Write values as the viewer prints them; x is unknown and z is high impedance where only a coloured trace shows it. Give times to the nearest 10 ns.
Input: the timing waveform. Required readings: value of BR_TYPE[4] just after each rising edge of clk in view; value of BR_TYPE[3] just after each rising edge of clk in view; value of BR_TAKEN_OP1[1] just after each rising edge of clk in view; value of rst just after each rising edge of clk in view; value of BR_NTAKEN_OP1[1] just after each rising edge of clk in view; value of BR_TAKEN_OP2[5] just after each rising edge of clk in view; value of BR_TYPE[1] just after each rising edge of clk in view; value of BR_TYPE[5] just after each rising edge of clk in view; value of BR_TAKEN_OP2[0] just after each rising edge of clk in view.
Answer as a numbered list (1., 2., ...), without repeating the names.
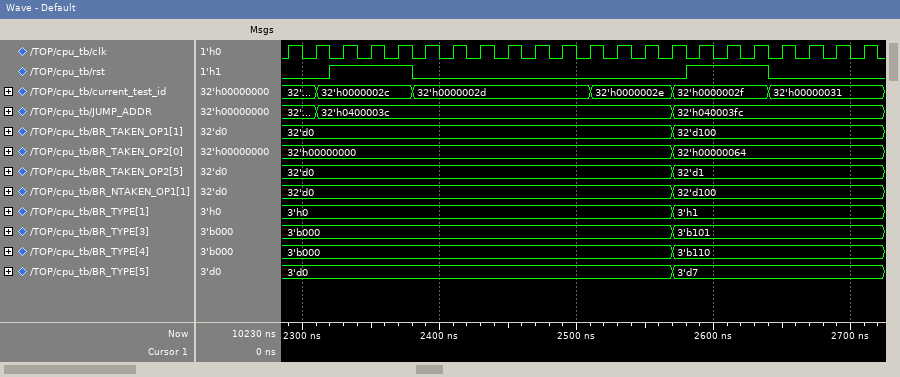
1. 3'b000, 3'b000, 3'b000, 3'b000, 3'b000, 3'b000, 3'b000, 3'b000, 3'b000, 3'b000, 3'b000, 3'b000, 3'b000, 3'b000, 3'b110, 3'b110, 3'b110, 3'b110, 3'b110, 3'b110, 3'b110, 3'b110
2. 3'b000, 3'b000, 3'b000, 3'b000, 3'b000, 3'b000, 3'b000, 3'b000, 3'b000, 3'b000, 3'b000, 3'b000, 3'b000, 3'b000, 3'b101, 3'b101, 3'b101, 3'b101, 3'b101, 3'b101, 3'b101, 3'b101
3. 32'd0, 32'd0, 32'd0, 32'd0, 32'd0, 32'd0, 32'd0, 32'd0, 32'd0, 32'd0, 32'd0, 32'd0, 32'd0, 32'd0, 32'd100, 32'd100, 32'd100, 32'd100, 32'd100, 32'd100, 32'd100, 32'd100
4. 0 0 1 1 1 0 0 0 0 0 0 0 0 0 0 1 1 1 0 0 0 0
5. 32'd0, 32'd0, 32'd0, 32'd0, 32'd0, 32'd0, 32'd0, 32'd0, 32'd0, 32'd0, 32'd0, 32'd0, 32'd0, 32'd0, 32'd100, 32'd100, 32'd100, 32'd100, 32'd100, 32'd100, 32'd100, 32'd100
6. 32'd0, 32'd0, 32'd0, 32'd0, 32'd0, 32'd0, 32'd0, 32'd0, 32'd0, 32'd0, 32'd0, 32'd0, 32'd0, 32'd0, 32'd1, 32'd1, 32'd1, 32'd1, 32'd1, 32'd1, 32'd1, 32'd1
7. 3'h0, 3'h0, 3'h0, 3'h0, 3'h0, 3'h0, 3'h0, 3'h0, 3'h0, 3'h0, 3'h0, 3'h0, 3'h0, 3'h0, 3'h1, 3'h1, 3'h1, 3'h1, 3'h1, 3'h1, 3'h1, 3'h1
8. 3'd0, 3'd0, 3'd0, 3'd0, 3'd0, 3'd0, 3'd0, 3'd0, 3'd0, 3'd0, 3'd0, 3'd0, 3'd0, 3'd0, 3'd7, 3'd7, 3'd7, 3'd7, 3'd7, 3'd7, 3'd7, 3'd7
9. 32'h00000000, 32'h00000000, 32'h00000000, 32'h00000000, 32'h00000000, 32'h00000000, 32'h00000000, 32'h00000000, 32'h00000000, 32'h00000000, 32'h00000000, 32'h00000000, 32'h00000000, 32'h00000000, 32'h00000064, 32'h00000064, 32'h00000064, 32'h00000064, 32'h00000064, 32'h00000064, 32'h00000064, 32'h00000064
